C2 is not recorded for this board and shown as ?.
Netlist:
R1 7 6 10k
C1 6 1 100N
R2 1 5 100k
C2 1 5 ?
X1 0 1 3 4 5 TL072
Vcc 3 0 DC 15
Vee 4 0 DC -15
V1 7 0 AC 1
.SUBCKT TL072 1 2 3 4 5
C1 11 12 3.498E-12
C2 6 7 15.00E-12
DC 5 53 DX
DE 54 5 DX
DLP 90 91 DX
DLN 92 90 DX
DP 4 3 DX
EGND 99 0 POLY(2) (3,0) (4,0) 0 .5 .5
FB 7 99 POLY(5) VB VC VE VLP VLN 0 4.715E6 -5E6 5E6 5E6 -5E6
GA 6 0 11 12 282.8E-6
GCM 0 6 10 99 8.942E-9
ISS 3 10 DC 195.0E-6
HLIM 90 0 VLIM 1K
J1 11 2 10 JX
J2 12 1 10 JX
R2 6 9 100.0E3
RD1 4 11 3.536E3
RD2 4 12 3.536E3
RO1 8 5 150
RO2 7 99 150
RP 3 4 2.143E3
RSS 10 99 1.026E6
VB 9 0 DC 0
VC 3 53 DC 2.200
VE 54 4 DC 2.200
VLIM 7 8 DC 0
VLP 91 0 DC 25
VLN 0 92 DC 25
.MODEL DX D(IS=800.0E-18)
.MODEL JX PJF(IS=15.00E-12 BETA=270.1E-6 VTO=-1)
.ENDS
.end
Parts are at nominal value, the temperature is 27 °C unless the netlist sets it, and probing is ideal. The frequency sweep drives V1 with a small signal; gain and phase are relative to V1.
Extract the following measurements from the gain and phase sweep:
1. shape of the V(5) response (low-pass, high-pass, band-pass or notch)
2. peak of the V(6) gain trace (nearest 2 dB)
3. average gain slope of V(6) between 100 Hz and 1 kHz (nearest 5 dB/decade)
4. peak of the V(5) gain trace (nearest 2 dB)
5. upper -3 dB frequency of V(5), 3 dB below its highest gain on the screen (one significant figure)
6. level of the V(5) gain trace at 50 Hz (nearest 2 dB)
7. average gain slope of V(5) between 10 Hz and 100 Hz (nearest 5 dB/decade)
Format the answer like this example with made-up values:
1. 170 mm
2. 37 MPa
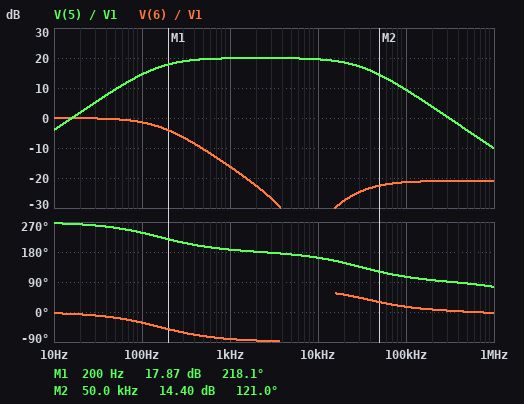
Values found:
1. band-pass
2. 0 dB
3. -15 dB/decade
4. 20 dB
5. 30 kHz
6. 10 dB
7. 20 dB/decade
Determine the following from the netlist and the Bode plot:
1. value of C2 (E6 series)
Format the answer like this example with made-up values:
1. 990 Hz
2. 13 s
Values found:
1. 47 pF
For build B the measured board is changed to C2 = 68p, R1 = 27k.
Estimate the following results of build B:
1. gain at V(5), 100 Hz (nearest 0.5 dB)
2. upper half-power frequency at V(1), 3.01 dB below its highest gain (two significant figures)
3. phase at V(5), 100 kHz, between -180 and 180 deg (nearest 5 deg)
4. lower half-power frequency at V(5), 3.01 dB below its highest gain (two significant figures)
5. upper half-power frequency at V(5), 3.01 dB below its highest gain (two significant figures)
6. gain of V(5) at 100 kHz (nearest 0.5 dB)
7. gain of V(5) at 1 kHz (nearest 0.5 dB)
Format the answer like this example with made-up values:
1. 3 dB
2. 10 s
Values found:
1. 10.0 dB
2. 6.4 MHz
3. 100 deg
4. 59 Hz
5. 23 kHz
6. -1.5 dB
7. 11.5 dB
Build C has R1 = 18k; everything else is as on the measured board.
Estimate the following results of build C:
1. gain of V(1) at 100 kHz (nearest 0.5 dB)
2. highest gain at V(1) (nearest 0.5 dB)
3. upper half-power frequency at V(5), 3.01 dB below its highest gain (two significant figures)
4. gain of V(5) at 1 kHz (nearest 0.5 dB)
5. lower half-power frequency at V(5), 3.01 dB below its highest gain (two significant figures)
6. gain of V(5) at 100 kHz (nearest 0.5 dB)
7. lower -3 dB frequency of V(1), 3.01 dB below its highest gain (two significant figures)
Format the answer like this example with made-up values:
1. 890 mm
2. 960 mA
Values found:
1. -26.0 dB
2. -25.0 dB
3. 32 kHz
4. 15.0 dB
5. 88 Hz
6. 4.5 dB
7. 36 kHz
